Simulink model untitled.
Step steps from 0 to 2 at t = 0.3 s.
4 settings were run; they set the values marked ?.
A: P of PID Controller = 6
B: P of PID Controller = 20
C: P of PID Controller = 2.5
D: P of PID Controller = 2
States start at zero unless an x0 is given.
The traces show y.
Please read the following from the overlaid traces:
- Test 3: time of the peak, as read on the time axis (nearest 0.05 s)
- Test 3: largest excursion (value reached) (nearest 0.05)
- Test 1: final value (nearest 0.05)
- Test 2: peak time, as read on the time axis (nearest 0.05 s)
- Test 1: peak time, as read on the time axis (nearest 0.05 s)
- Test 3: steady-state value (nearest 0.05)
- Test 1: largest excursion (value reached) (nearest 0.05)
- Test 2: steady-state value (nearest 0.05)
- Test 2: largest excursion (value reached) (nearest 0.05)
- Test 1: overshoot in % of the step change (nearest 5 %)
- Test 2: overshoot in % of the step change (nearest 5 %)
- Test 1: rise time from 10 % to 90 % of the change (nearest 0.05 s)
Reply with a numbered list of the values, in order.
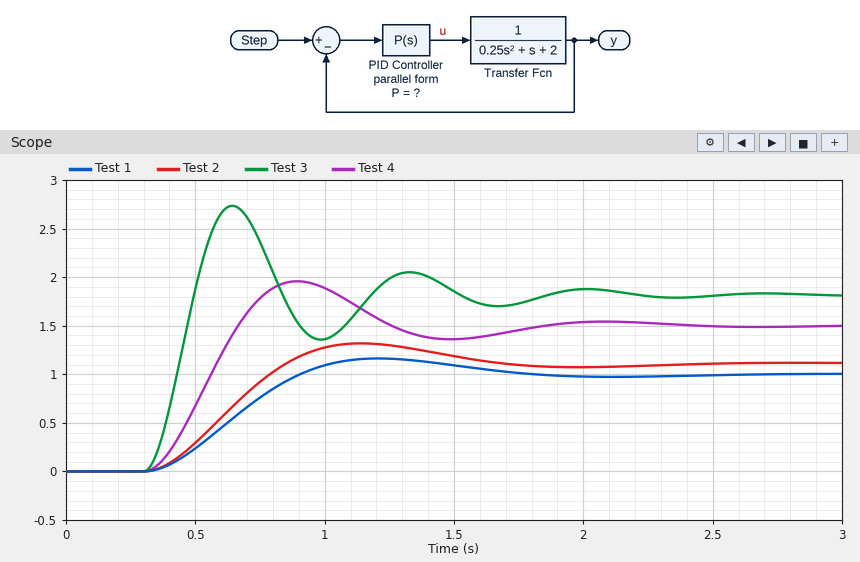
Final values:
1. 0.65 s
2. 2.75
3. 1.00
4. 1.15 s
5. 1.20 s
6. 1.80
7. 1.15
8. 1.10
9. 1.30
10. 15 %
11. 20 %
12. 0.40 s
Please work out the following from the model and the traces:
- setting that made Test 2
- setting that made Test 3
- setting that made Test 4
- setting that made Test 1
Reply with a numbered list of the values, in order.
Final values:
1. C
2. B
3. A
4. D
